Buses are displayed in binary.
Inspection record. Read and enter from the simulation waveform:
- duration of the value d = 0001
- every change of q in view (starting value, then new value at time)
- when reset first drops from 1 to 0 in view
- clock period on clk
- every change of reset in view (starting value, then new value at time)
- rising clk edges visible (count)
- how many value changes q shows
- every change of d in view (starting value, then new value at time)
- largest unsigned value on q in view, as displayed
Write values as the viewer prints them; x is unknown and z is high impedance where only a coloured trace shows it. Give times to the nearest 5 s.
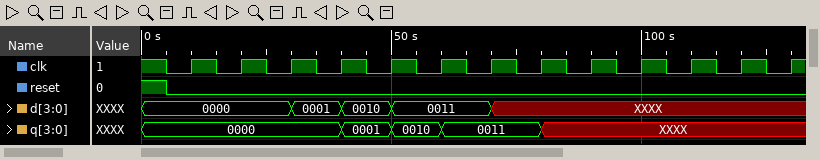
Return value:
10 s
0000, 0001 at 40 s, 0010 at 50 s, 0011 at 60 s, XXXX at 80 s
5 s
10 s
1, 0 at 5 s
13
4
0000, 0001 at 30 s, 0010 at 40 s, 0011 at 50 s, XXXX at 70 s
0011
